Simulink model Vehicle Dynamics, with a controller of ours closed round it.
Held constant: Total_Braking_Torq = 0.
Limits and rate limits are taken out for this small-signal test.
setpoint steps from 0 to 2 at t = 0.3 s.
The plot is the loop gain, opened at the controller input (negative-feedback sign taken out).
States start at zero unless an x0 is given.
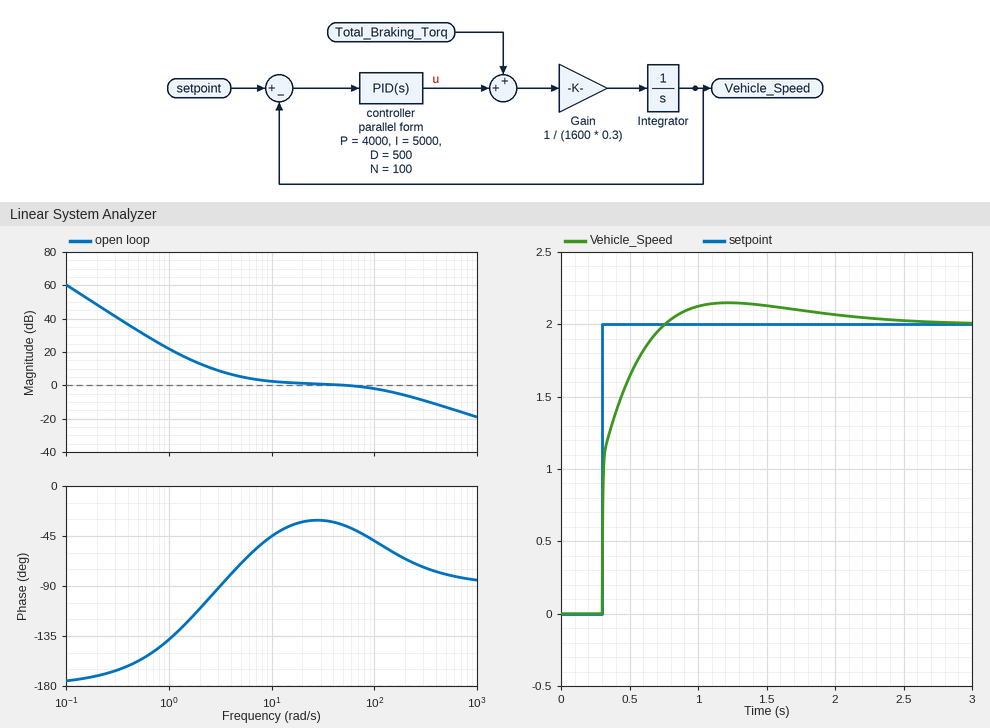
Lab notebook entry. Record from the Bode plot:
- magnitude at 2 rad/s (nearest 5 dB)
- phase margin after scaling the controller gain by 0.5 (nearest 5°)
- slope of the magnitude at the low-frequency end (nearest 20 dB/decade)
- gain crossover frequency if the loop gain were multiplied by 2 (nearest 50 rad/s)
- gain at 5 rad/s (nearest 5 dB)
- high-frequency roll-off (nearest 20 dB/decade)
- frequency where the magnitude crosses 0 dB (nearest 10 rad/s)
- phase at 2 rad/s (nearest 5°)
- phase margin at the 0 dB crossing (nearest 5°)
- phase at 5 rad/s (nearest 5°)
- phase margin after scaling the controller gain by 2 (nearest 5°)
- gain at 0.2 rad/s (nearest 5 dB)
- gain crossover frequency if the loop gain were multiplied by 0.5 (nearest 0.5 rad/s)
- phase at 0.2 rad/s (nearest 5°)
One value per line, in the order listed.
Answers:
15 dB
105°
-40 dB/decade
200 rad/s
5 dB
-20 dB/decade
50 rad/s
-110°
145°
-70°
115°
50 dB
4.5 rad/s
-170°
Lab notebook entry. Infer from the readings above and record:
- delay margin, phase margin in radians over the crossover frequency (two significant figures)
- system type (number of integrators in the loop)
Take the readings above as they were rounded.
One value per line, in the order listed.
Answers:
0.051 s
2
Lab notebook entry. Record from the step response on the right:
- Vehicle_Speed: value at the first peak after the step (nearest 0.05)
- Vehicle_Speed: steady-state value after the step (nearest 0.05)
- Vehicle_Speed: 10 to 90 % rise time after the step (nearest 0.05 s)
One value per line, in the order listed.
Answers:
2.15
2.00
0.30 s
